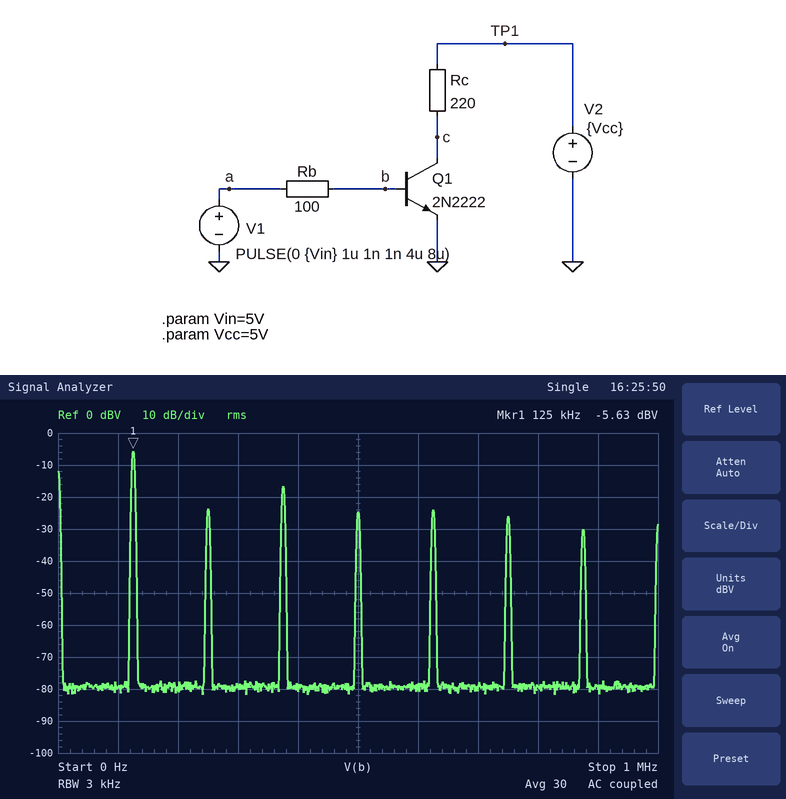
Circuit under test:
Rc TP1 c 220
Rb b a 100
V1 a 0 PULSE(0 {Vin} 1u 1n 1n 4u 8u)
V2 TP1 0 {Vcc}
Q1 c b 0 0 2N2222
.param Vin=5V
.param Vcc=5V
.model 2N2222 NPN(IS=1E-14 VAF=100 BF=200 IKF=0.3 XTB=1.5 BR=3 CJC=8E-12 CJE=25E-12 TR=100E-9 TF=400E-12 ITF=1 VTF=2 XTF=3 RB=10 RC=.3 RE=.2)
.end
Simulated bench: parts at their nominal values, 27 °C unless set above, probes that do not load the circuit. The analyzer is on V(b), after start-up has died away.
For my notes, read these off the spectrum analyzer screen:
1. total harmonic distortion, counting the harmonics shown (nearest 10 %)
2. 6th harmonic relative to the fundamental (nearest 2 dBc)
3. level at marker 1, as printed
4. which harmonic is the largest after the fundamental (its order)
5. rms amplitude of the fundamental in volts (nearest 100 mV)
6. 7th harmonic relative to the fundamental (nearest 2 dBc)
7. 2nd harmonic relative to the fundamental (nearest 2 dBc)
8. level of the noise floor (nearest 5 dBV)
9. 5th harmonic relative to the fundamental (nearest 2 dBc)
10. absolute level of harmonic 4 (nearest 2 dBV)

40 %
-20 dBc
-5.63 dBV
3
500 mV
-24 dBc
-18 dBc
-80 dBV
-18 dBc
-24 dBV
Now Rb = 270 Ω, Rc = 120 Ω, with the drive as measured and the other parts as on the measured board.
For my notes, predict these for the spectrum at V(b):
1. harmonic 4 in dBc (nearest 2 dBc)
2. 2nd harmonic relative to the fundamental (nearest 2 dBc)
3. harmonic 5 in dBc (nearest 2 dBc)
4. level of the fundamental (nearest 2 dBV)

-16 dBc
-16 dBc
-20 dBc
-8 dBV
